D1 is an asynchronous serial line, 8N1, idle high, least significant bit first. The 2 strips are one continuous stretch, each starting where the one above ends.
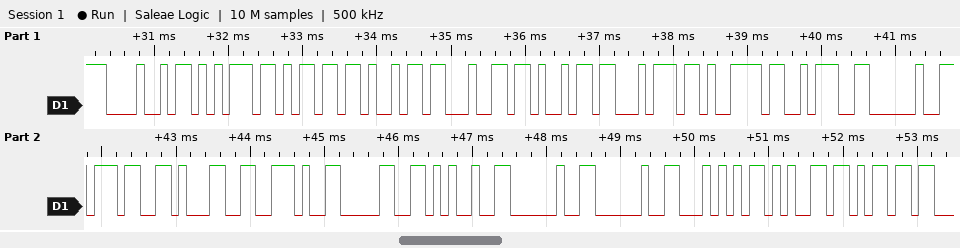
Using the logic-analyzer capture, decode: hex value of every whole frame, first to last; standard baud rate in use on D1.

48 75 6D 69 64 69 74 79 3A 20 37 31 2E 30 25 20 20 54 65 6D
9600 baud
